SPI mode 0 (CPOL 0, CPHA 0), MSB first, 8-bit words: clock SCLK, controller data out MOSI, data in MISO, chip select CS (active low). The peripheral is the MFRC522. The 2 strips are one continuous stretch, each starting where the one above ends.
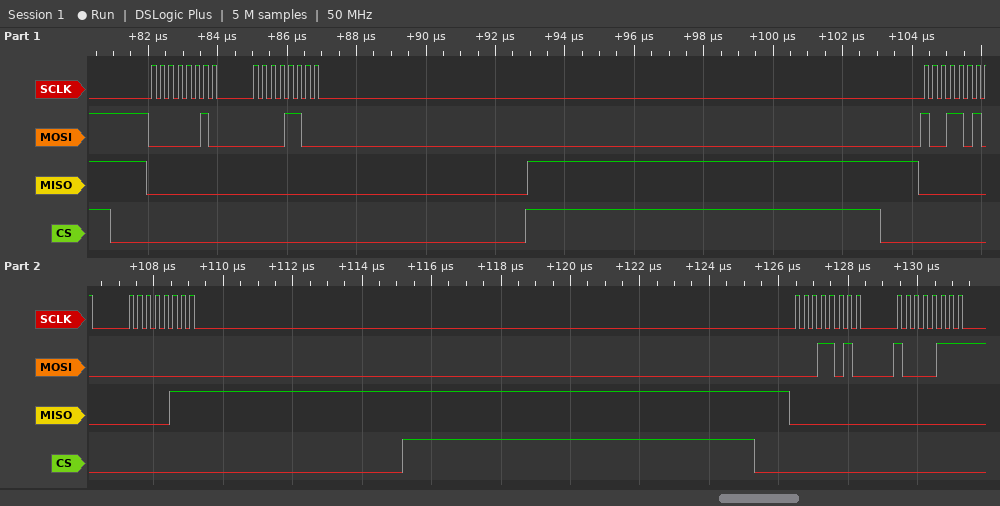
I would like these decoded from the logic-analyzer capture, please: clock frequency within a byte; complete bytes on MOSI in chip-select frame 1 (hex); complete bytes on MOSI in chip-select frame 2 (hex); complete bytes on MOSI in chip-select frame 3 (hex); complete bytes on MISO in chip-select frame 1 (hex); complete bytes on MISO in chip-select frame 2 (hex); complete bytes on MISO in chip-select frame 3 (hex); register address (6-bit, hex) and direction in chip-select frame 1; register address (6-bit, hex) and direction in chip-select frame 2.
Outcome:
4 MHz
0x02 0x0C
0x9A 0x00
0x1A 0x87
0x00 0x00
0x00 0x07
0x00 0x00
0x01 write
0x0D read
